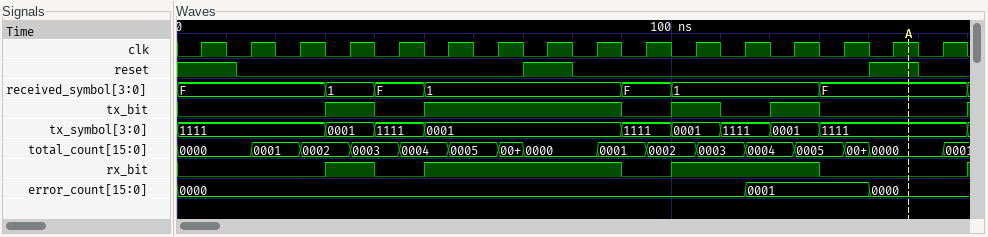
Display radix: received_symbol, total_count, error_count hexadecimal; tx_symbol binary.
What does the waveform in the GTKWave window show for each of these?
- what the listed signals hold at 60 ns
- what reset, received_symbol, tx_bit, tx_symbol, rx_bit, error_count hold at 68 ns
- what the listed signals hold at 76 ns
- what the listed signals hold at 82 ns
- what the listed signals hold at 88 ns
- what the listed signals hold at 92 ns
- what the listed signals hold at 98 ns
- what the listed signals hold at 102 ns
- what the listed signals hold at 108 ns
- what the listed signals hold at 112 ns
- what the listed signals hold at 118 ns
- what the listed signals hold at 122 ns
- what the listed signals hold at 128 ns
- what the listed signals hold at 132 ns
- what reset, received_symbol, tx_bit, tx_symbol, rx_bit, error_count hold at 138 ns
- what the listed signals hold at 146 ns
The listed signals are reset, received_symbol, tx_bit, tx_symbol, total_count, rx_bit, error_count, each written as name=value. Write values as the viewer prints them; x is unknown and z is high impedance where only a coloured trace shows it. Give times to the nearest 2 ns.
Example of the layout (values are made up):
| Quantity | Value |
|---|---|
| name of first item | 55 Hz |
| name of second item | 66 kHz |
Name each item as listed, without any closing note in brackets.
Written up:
| Quantity | Value |
|---|---|
| what the listed signals hold at 60 ns | reset=0, received_symbol=1, tx_bit=1, tx_symbol=0001, total_count=0005, rx_bit=1, error_count=0000 |
| what reset, received_symbol, tx_bit, tx_symbol, rx_bit, error_count hold at 68 ns | reset=0, received_symbol=1, tx_bit=1, tx_symbol=0001, rx_bit=1, error_count=0000 |
| what the listed signals hold at 76 ns | reset=1, received_symbol=1, tx_bit=1, tx_symbol=0001, total_count=0000, rx_bit=1, error_count=0000 |
| what the listed signals hold at 82 ns | reset=0, received_symbol=1, tx_bit=1, tx_symbol=0001, total_count=0000, rx_bit=1, error_count=0000 |
| what the listed signals hold at 88 ns | reset=0, received_symbol=1, tx_bit=1, tx_symbol=0001, total_count=0001, rx_bit=1, error_count=0000 |
| what the listed signals hold at 92 ns | reset=0, received_symbol=F, tx_bit=0, tx_symbol=1111, total_count=0001, rx_bit=0, error_count=0000 |
| what the listed signals hold at 98 ns | reset=0, received_symbol=F, tx_bit=0, tx_symbol=1111, total_count=0002, rx_bit=0, error_count=0000 |
| what the listed signals hold at 102 ns | reset=0, received_symbol=1, tx_bit=1, tx_symbol=0001, total_count=0002, rx_bit=1, error_count=0000 |
| what the listed signals hold at 108 ns | reset=0, received_symbol=1, tx_bit=1, tx_symbol=0001, total_count=0003, rx_bit=1, error_count=0000 |
| what the listed signals hold at 112 ns | reset=0, received_symbol=1, tx_bit=0, tx_symbol=1111, total_count=0003, rx_bit=1, error_count=0000 |
| what the listed signals hold at 118 ns | reset=0, received_symbol=1, tx_bit=0, tx_symbol=1111, total_count=0004, rx_bit=1, error_count=0001 |
| what the listed signals hold at 122 ns | reset=0, received_symbol=1, tx_bit=1, tx_symbol=0001, total_count=0004, rx_bit=1, error_count=0001 |
| what the listed signals hold at 128 ns | reset=0, received_symbol=1, tx_bit=1, tx_symbol=0001, total_count=0005, rx_bit=1, error_count=0001 |
| what the listed signals hold at 132 ns | reset=0, received_symbol=F, tx_bit=0, tx_symbol=1111, total_count=0005, rx_bit=0, error_count=0001 |
| what reset, received_symbol, tx_bit, tx_symbol, rx_bit, error_count hold at 138 ns | reset=0, received_symbol=F, tx_bit=0, tx_symbol=1111, rx_bit=0, error_count=0001 |
| what the listed signals hold at 146 ns | reset=1, received_symbol=F, tx_bit=0, tx_symbol=1111, total_count=0000, rx_bit=0, error_count=0000 |
